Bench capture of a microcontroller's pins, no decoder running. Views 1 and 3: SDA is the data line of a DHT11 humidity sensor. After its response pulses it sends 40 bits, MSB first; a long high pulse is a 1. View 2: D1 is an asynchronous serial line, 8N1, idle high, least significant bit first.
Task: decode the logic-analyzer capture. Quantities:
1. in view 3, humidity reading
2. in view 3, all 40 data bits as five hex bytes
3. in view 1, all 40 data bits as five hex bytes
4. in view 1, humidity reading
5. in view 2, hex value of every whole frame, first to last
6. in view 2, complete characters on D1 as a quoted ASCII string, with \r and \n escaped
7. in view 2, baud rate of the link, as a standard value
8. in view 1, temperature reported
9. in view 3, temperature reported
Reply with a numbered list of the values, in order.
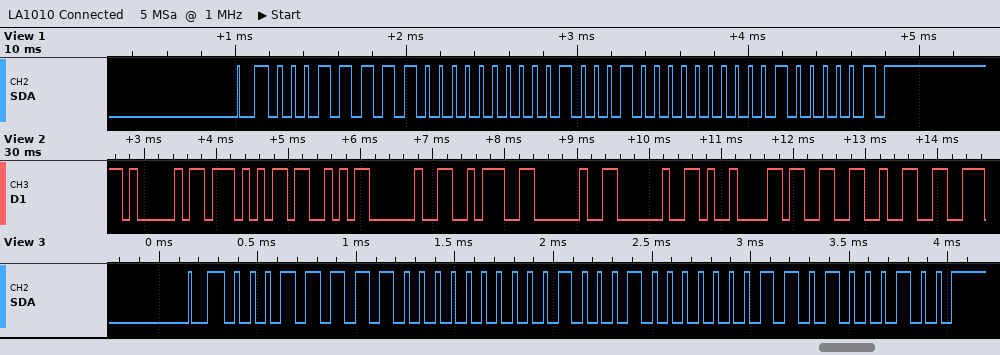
1. 31 %
2. 1F 00 22 03 44
3. 1F 00 22 00 41
4. 31 %
5. 0x41 0x57 0x53 0x20 0x3A 0x20 0x20 0x09 0x33 0x32
6. "AWS :  \t32"
7. 9600 baud
8. 34.0 °C
9. 34.3 °C
